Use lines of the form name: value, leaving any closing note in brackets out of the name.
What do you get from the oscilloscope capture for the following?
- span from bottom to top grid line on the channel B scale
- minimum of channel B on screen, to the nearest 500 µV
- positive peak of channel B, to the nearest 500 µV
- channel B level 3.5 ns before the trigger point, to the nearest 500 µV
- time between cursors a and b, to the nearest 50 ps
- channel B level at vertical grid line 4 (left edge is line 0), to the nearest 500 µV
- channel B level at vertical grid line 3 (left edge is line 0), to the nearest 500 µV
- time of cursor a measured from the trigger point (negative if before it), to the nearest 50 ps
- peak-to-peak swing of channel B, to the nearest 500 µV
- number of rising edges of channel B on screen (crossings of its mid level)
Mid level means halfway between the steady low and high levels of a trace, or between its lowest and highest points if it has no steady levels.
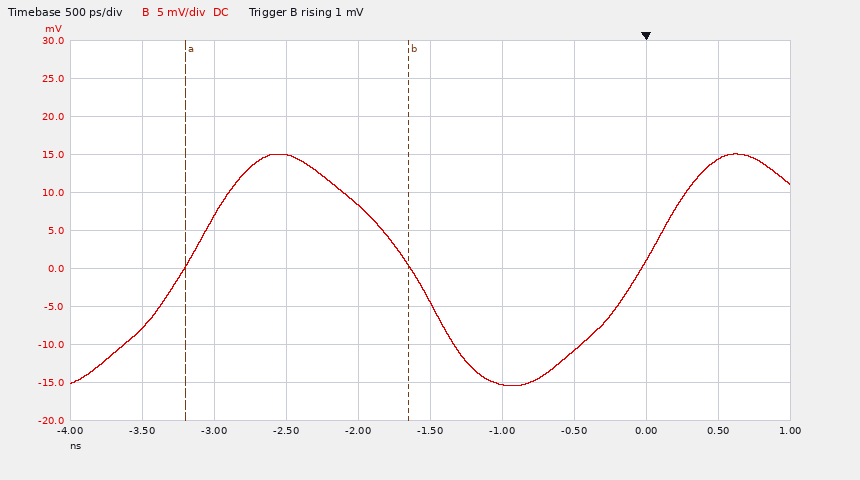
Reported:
span from bottom to top grid line on the channel B scale: 50 mV
minimum of channel B on screen, to the nearest 500 µV: -15.5 mV
positive peak of channel B, to the nearest 500 µV: 15.0 mV
channel B level 3.5 ns before the trigger point, to the nearest 500 µV: -8.0 mV
time between cursors a and b, to the nearest 50 ps: 1.55 ns
channel B level at vertical grid line 4 (left edge is line 0), to the nearest 500 µV: 8.5 mV
channel B level at vertical grid line 3 (left edge is line 0), to the nearest 500 µV: 15.0 mV
time of cursor a measured from the trigger point (negative if before it), to the nearest 50 ps: -3.20 ns
peak-to-peak swing of channel B, to the nearest 500 µV: 30.5 mV
number of rising edges of channel B on screen: 2
